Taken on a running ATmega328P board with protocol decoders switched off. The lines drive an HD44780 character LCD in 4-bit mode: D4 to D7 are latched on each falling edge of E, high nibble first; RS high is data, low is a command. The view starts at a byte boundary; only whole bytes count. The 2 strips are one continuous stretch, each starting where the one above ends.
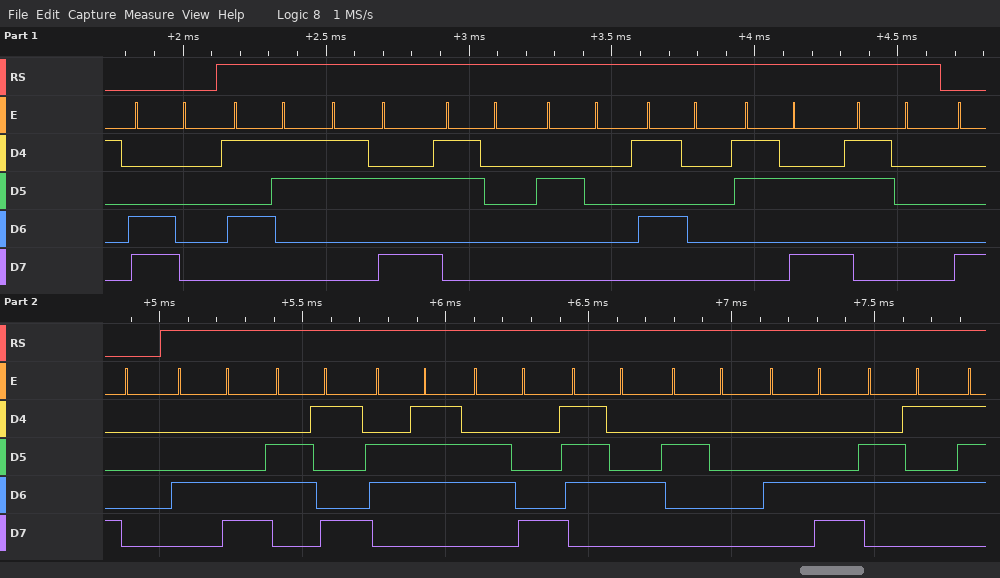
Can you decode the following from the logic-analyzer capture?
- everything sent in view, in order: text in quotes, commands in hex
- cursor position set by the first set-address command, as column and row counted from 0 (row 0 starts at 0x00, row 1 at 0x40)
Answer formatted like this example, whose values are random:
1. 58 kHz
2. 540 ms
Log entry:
1. 0xC0 "S:0 P:0" 0x80 "Light Le"
2. column 0, row 1
